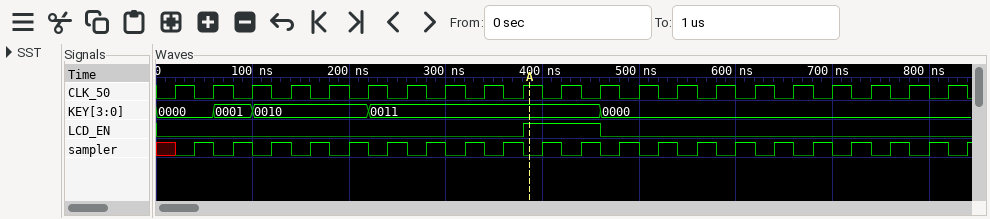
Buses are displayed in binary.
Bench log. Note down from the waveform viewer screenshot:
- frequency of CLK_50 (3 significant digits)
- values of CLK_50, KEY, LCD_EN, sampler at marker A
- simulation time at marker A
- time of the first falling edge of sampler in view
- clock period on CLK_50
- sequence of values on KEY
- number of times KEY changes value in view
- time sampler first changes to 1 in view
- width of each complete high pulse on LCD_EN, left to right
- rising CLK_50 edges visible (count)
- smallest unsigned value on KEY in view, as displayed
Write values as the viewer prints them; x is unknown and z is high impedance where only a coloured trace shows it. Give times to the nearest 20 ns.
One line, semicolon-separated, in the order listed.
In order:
25.0 MHz; CLK_50=1, KEY=0011, LCD_EN=1, sampler=0; 380 ns; 60 ns; 40 ns; 0000, 0001, 0010, 0011, 0000; 4; 40 ns; 80 ns; 21; 0000
